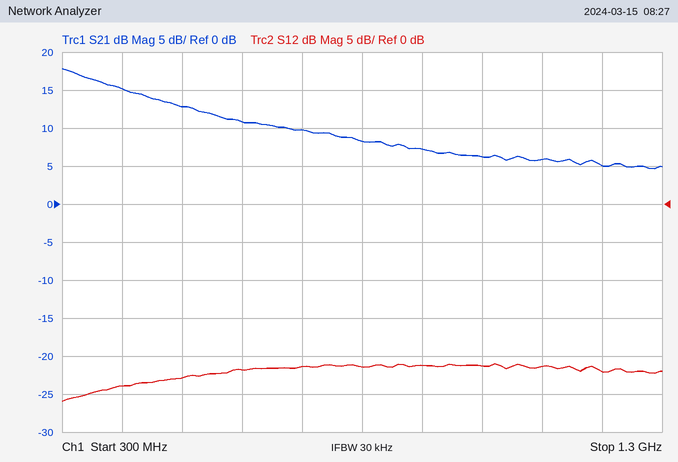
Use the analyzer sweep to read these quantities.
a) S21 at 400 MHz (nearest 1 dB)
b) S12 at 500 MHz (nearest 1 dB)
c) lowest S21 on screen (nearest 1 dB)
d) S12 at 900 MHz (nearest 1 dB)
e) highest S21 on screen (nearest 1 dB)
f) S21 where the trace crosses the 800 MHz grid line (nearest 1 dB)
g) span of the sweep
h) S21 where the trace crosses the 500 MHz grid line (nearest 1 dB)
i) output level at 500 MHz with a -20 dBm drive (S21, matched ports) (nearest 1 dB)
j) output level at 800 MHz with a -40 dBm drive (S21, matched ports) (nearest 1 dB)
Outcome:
15 dB
-23 dB
5 dB
-21 dB
18 dB
8 dB
1 GHz
13 dB
-7 dBm
-32 dBm
